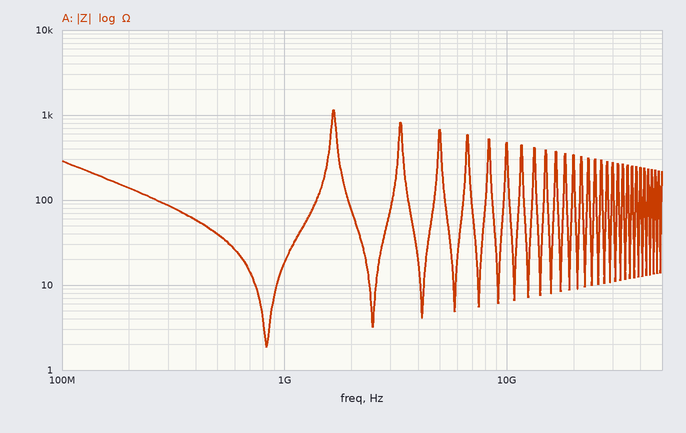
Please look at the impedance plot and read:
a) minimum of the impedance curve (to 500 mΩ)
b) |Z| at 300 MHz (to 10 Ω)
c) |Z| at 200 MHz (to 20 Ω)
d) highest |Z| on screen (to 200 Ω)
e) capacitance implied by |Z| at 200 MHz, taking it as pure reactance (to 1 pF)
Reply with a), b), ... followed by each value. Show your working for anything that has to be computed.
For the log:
a) 2.0 Ω
b) 90 Ω
c) 140 Ω
d) 1.2 kΩ
e) C = 1/(2π × 200 MHz × 140 Ω) ≈ 6 pF
